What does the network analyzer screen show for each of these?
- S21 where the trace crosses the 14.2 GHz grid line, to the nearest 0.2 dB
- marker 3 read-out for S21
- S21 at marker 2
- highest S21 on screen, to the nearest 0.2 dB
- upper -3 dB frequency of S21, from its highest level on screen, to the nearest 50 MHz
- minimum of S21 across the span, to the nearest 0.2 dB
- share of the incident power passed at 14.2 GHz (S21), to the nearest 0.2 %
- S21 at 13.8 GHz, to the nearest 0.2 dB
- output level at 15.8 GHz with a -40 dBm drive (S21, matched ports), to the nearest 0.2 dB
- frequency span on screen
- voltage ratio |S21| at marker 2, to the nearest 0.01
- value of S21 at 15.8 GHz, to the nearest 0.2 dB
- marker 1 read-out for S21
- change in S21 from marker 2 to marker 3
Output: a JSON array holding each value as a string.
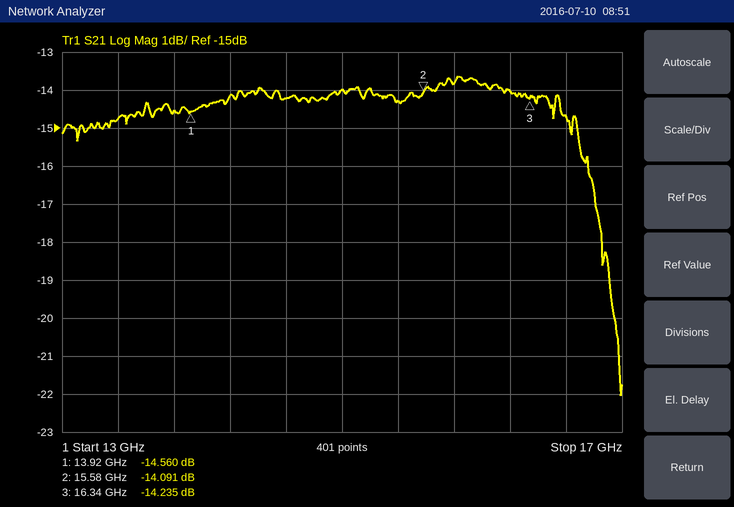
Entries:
["-14.2 dB", "-14.235 dB", "-14.091 dB", "-13.6 dB", "16.80 GHz", "-22.0 dB", "3.8 %", "-14.6 dB", "-53.8 dBm", "4 GHz", "0.20", "-13.8 dB", "-14.560 dB", "-0.144 dB"]
